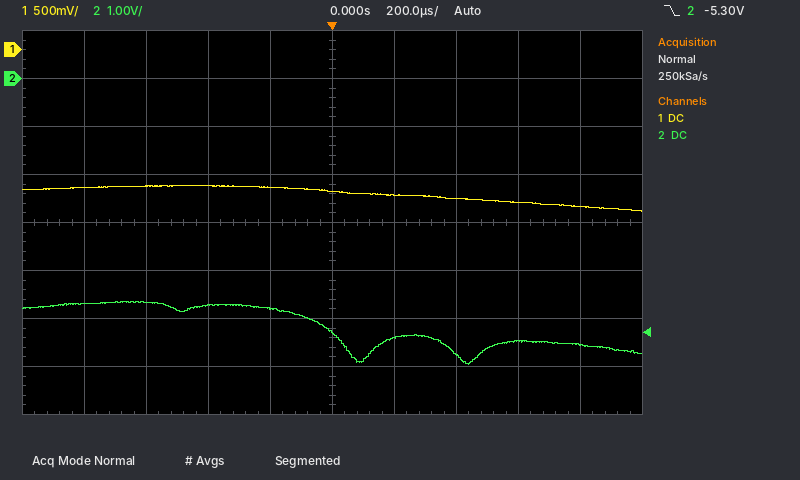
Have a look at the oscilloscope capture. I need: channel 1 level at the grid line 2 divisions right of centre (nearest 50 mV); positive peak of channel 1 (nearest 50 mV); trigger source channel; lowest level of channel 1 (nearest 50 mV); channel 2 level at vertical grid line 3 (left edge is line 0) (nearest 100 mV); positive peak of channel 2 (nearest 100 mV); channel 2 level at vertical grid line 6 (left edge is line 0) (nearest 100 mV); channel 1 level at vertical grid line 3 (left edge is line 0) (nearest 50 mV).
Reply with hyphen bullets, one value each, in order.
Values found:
- -1.55 V
- -1.40 V
- channel 2
- -1.70 V
- -4.7 V
- -4.6 V
- -5.4 V
- -1.40 V
